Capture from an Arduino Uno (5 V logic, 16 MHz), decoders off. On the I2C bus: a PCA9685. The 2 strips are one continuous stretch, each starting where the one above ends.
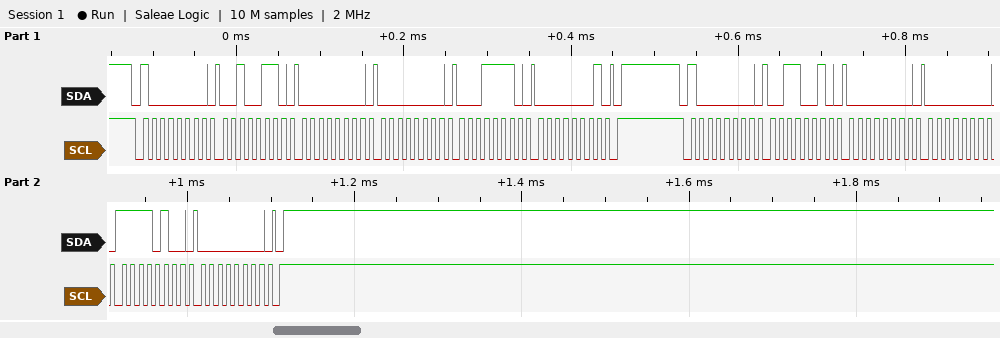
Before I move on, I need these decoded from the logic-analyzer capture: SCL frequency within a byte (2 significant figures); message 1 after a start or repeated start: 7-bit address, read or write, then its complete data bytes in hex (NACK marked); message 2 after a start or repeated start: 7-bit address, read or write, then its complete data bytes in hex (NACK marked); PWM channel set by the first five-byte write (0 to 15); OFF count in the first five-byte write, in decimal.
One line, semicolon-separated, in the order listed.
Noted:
100 kHz; 0x40 write: 26 00 00 1E 01; 0x40 write: 32 00 00 F4 00; 8; 286
